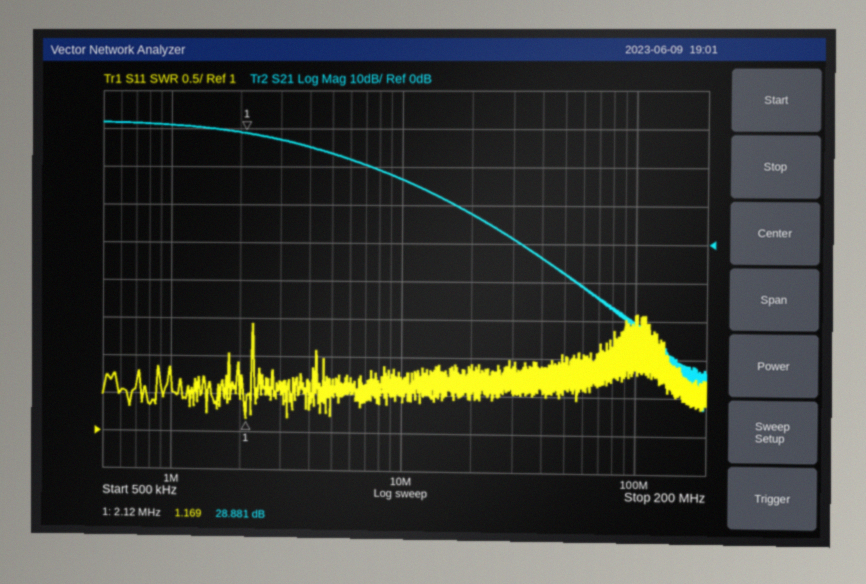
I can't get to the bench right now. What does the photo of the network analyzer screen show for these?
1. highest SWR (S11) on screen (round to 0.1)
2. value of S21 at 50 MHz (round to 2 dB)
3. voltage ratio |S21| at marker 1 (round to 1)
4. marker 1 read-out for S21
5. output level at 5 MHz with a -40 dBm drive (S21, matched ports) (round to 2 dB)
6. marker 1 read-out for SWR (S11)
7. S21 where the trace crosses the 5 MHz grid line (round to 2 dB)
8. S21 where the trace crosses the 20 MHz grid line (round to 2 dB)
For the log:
2.6
-8 dB
28
28.881 dB
-16 dBm
1.169
24 dB
8 dB
